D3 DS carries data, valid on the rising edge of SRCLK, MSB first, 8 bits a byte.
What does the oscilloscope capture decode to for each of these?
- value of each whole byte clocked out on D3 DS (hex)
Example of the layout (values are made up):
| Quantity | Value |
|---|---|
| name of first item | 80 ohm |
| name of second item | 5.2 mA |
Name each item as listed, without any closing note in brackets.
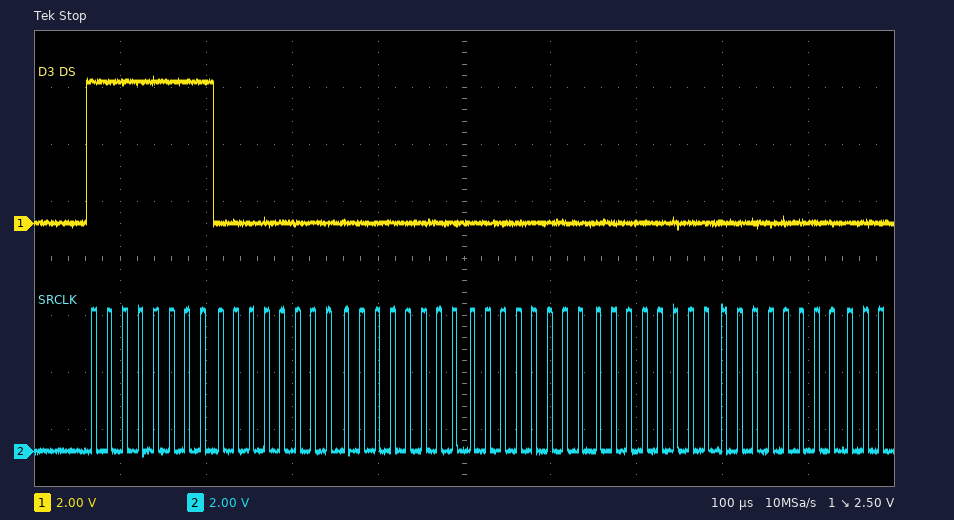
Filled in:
| Quantity | Value |
|---|---|
| value of each whole byte clocked out on D3 DS | FF 00 00 00 00 00 |
